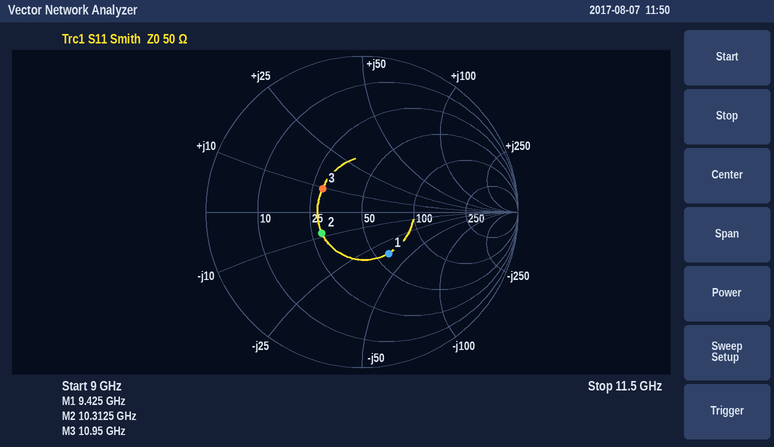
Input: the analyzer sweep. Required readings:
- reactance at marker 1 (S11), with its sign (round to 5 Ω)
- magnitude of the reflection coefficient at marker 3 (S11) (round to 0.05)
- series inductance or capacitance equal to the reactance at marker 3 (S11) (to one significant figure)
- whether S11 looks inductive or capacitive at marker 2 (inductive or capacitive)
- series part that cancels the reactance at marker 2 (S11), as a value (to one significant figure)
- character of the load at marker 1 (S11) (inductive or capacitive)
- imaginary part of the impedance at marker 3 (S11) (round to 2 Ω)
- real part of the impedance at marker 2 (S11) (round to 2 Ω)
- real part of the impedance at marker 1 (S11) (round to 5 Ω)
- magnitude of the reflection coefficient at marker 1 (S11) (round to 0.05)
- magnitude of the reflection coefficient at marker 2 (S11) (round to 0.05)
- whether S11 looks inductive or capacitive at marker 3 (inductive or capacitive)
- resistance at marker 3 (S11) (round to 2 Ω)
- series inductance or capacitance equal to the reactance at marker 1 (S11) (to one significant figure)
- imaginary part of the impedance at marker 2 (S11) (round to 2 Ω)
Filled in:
-35 Ω
0.30
100 pH
capacitive
100 pH
capacitive
+10 Ω
28 Ω
60 Ω
0.30
0.30
inductive
28 Ω
500 fF
-8 Ω
